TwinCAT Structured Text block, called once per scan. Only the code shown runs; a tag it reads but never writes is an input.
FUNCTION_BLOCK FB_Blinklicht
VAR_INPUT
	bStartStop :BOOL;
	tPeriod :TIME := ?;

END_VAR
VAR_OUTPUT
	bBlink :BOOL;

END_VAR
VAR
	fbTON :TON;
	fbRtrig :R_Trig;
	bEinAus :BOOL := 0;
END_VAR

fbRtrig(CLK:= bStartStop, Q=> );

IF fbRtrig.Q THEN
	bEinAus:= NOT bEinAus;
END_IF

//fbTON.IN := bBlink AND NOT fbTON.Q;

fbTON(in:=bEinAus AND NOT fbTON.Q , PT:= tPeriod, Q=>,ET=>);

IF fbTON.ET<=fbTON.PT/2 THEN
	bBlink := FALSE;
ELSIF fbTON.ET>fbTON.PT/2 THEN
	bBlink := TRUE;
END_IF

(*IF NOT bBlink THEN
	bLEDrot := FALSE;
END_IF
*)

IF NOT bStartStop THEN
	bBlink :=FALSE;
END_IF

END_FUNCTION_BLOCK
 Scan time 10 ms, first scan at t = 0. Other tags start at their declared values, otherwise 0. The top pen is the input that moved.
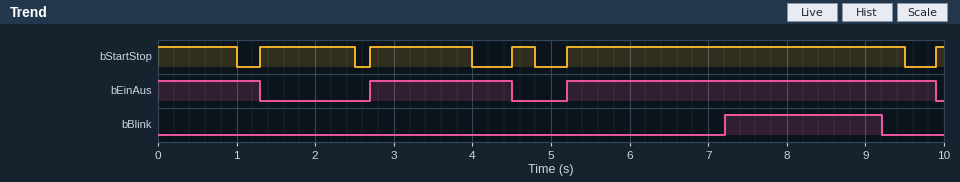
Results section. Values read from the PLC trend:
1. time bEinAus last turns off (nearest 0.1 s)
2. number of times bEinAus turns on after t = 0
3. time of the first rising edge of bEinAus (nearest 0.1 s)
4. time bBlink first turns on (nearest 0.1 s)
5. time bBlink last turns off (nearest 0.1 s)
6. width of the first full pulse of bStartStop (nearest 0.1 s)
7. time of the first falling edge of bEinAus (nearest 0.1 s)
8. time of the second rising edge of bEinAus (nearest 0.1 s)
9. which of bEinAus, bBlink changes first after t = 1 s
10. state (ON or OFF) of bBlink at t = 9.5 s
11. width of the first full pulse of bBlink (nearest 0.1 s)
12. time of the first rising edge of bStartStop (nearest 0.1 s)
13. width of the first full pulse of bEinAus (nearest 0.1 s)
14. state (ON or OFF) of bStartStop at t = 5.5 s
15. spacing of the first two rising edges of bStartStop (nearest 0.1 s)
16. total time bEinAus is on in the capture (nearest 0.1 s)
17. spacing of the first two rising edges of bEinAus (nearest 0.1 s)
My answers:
9.9 s
2
2.7 s
7.2 s
9.2 s
1.2 s
1.3 s
5.2 s
bEinAus
OFF
2.0 s
1.3 s
1.8 s
ON
1.4 s
7.8 s
2.5 s
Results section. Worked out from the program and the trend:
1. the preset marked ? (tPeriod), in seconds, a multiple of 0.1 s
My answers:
4.0 s
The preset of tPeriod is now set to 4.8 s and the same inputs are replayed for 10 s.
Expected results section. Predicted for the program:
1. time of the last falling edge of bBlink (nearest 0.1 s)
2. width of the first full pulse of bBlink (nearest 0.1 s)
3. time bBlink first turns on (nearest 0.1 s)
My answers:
9.5 s
1.9 s
7.6 s
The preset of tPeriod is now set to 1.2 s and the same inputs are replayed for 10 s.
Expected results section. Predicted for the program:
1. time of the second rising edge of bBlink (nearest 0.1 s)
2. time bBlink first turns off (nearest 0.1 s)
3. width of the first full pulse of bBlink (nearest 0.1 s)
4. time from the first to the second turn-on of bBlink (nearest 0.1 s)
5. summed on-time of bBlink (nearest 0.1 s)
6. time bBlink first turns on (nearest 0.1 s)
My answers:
3.3 s
1.0 s
0.4 s
2.7 s
2.8 s
0.6 s
